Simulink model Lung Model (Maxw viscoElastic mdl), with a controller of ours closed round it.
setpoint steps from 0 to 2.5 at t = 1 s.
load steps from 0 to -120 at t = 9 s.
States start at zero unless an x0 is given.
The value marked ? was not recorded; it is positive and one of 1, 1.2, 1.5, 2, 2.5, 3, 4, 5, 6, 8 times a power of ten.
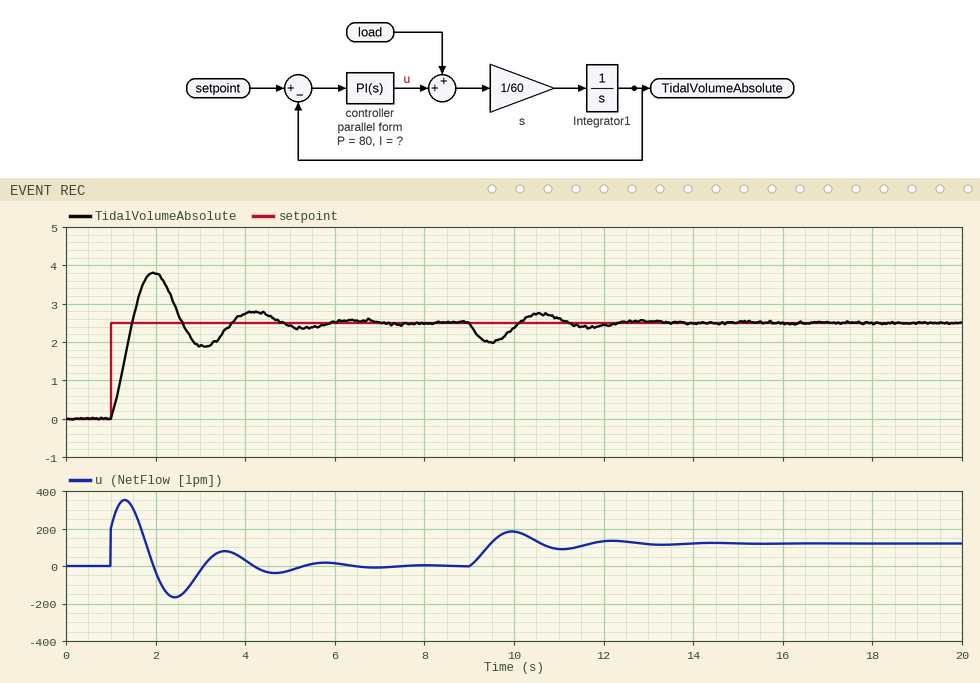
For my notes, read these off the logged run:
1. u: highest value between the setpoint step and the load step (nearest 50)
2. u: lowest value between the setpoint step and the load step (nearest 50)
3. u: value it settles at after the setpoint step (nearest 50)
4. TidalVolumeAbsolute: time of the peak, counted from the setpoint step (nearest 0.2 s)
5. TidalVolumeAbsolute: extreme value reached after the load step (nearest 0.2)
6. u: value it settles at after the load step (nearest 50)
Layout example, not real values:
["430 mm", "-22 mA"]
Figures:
["350", "-150", "0", "1.0 s", "2.0", "100"]
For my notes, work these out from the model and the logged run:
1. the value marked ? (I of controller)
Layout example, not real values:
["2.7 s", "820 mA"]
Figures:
["500"]
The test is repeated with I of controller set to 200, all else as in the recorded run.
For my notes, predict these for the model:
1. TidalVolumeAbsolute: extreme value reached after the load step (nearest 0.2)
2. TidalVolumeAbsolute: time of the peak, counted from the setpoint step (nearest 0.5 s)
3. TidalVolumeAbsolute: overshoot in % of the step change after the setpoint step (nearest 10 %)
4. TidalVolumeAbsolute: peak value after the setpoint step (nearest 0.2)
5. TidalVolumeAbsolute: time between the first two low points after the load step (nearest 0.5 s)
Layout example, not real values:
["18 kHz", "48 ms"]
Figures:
["1.8", "1.5 s", "40 %", "3.4", "3.5 s"]
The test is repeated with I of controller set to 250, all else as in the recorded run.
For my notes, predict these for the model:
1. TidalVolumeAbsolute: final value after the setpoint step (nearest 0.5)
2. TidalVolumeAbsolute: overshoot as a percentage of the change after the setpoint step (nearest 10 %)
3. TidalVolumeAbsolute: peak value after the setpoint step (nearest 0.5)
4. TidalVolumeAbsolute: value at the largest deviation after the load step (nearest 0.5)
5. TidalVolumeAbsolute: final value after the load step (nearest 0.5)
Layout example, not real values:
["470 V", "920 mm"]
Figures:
["2.5", "40 %", "3.5", "2.0", "2.5"]
